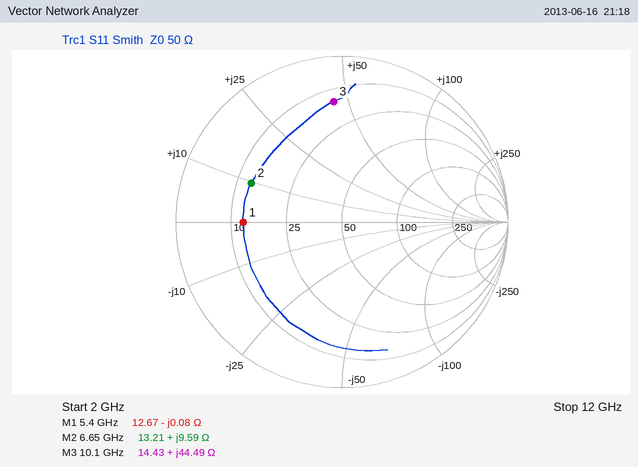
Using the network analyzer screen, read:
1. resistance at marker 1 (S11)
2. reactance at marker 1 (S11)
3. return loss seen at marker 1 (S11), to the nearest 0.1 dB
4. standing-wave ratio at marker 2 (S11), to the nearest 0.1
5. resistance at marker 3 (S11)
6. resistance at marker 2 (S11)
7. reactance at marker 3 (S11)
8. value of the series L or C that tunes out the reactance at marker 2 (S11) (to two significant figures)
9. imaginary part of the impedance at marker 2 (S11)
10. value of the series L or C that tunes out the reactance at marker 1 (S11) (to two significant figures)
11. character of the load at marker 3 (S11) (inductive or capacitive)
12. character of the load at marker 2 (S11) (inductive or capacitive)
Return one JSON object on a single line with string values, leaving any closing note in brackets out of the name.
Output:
{"resistance at marker 1": "12.67 Ω", "reactance at marker 1": "-0.08 Ω", "return loss seen at marker 1 (S11), to the nearest 0.1 dB": "4.5 dB", "standing-wave ratio at marker 2 (S11), to the nearest 0.1": "3.9", "resistance at marker 3": "14.43 Ω", "resistance at marker 2": "13.21 Ω", "reactance at marker 3": "+44.49 Ω", "value of the series L or C that tunes out the reactance at marker 2 (S11)": "2.5 pF", "imaginary part of the impedance at marker 2": "+9.59 Ω", "value of the series L or C that tunes out the reactance at marker 1 (S11)": "2.4 pH", "character of the load at marker 3 (S11)": "inductive", "character of the load at marker 2 (S11)": "inductive"}
